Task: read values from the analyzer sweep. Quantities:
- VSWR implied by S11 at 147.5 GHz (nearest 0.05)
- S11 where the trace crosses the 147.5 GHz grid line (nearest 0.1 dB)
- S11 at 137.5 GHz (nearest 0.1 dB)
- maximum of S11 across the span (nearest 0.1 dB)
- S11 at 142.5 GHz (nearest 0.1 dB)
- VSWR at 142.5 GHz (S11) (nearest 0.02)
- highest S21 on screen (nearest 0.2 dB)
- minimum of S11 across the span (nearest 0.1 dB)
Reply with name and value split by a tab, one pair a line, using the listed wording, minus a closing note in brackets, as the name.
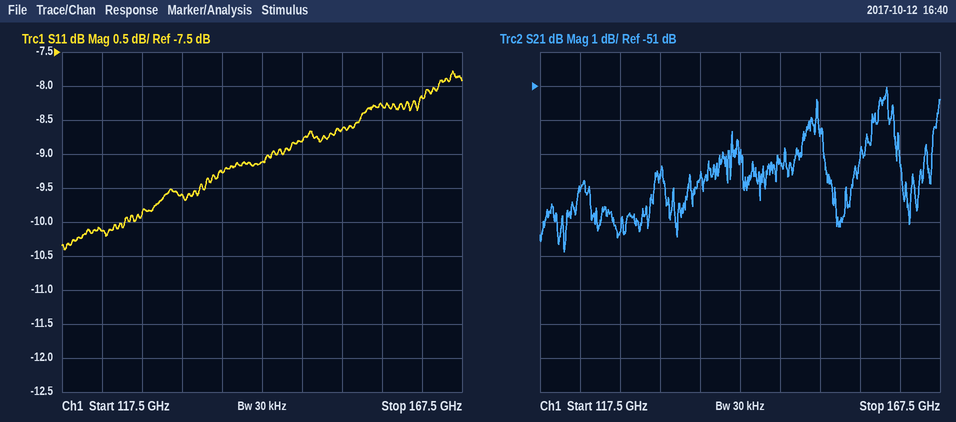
VSWR implied by S11 at 147.5 GHz	2.15
S11 where the trace crosses the 147.5 GHz grid line	-8.8 dB
S11 at 137.5 GHz	-9.3 dB
maximum of S11 across the span	-7.8 dB
S11 at 142.5 GHz	-9.1 dB
VSWR at 142.5 GHz (S11)	2.08
highest S21 on screen	-51.0 dB
minimum of S11 across the span	-10.4 dB
